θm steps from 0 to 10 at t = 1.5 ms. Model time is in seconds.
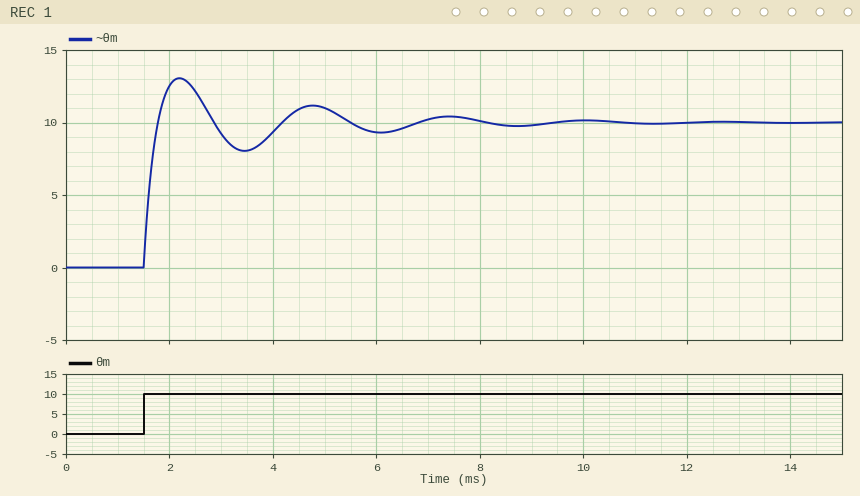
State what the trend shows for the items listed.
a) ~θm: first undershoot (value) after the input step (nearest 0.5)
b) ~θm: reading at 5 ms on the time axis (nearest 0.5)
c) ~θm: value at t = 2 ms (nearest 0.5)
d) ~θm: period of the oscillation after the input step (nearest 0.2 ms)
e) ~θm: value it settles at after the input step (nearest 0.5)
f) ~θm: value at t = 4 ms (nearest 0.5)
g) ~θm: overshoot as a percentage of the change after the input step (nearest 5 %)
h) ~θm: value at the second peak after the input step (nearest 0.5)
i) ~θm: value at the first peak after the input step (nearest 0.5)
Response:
8.0
11.0
12.5
2.6 ms
10.0
9.5
30 %
11.0
13.0
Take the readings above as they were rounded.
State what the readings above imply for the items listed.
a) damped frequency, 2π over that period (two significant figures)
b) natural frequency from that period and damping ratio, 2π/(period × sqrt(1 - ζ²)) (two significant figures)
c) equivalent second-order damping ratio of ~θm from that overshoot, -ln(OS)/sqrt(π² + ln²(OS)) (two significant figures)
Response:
2.4 rad/ms
2.6 rad/ms
0.36
